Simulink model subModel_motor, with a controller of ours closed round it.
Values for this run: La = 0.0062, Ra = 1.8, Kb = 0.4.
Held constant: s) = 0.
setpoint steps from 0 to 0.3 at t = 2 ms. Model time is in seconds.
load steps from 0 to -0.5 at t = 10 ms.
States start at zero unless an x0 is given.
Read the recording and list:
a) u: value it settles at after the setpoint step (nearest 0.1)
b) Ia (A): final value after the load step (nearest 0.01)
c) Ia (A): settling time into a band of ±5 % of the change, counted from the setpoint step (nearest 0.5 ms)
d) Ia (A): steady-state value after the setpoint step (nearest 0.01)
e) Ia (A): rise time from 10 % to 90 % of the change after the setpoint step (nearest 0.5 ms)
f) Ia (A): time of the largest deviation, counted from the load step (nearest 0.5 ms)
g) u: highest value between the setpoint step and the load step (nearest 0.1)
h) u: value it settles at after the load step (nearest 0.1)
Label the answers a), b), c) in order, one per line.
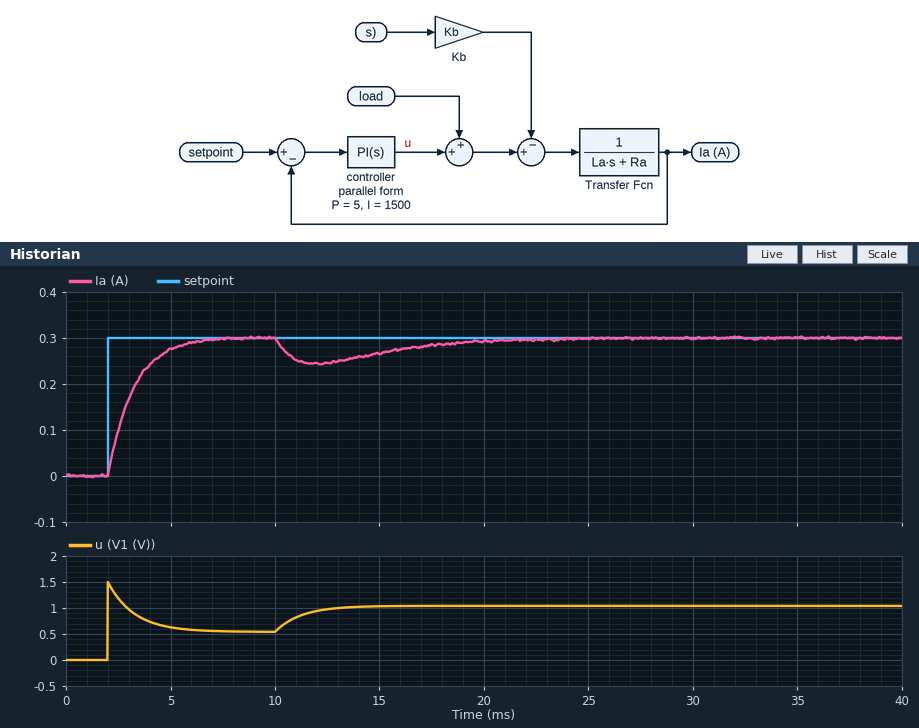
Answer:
a) 0.5
b) 0.30
c) 3.5 ms
d) 0.30
e) 2.5 ms
f) 2.0 ms
g) 1.5
h) 1.0
